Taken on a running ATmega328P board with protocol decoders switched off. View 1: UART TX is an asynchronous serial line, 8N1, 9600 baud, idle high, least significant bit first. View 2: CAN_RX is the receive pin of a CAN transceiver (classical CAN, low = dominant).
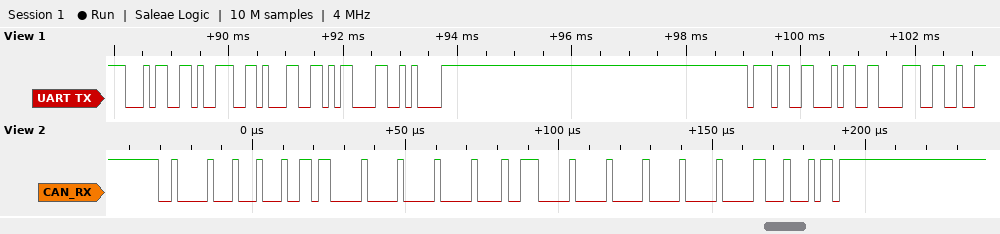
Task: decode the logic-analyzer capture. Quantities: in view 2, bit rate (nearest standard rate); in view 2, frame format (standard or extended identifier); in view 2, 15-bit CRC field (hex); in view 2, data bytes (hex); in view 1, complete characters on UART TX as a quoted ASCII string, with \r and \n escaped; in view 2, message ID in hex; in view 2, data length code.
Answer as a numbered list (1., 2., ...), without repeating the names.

1. 500 kbit/s
2. standard
3. 0x0445
4. 9B 00 00 00 9C 00 00 00
5. "491\r\n748"
6. 0x201
7. 8
